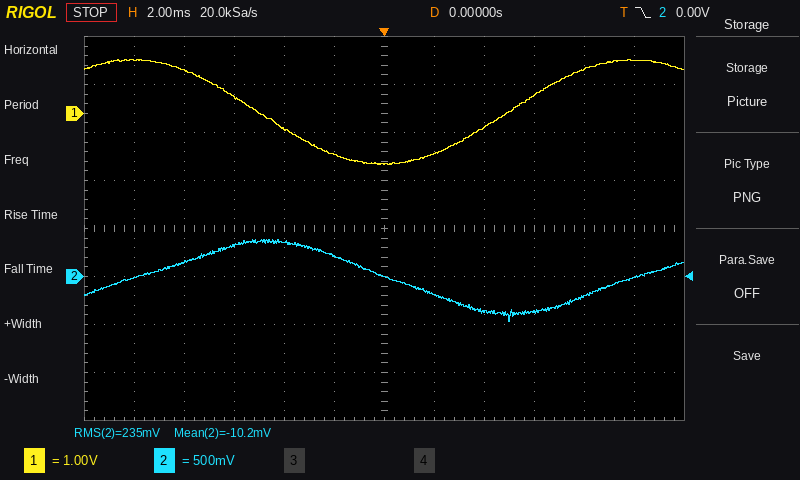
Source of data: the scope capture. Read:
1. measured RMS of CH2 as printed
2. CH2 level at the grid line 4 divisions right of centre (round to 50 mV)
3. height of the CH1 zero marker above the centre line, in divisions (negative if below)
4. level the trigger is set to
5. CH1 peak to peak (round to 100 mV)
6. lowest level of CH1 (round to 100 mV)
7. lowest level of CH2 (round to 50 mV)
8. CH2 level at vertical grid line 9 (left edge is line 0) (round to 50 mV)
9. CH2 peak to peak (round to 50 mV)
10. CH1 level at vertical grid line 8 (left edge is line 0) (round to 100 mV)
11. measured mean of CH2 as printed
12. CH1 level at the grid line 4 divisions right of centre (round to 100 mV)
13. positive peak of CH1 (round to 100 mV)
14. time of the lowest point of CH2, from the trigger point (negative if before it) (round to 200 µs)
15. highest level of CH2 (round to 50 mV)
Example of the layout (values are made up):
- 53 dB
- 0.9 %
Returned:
- 235 mV
- -200 mV
- +2.4 div
- 0.00 V
- 2.2 V
- -1.1 V
- -450 mV
- -350 mV
- 850 mV
- -300 mV
- -10.2 mV
- 900 mV
- 1.1 V
- +5.0 ms
- 400 mV
